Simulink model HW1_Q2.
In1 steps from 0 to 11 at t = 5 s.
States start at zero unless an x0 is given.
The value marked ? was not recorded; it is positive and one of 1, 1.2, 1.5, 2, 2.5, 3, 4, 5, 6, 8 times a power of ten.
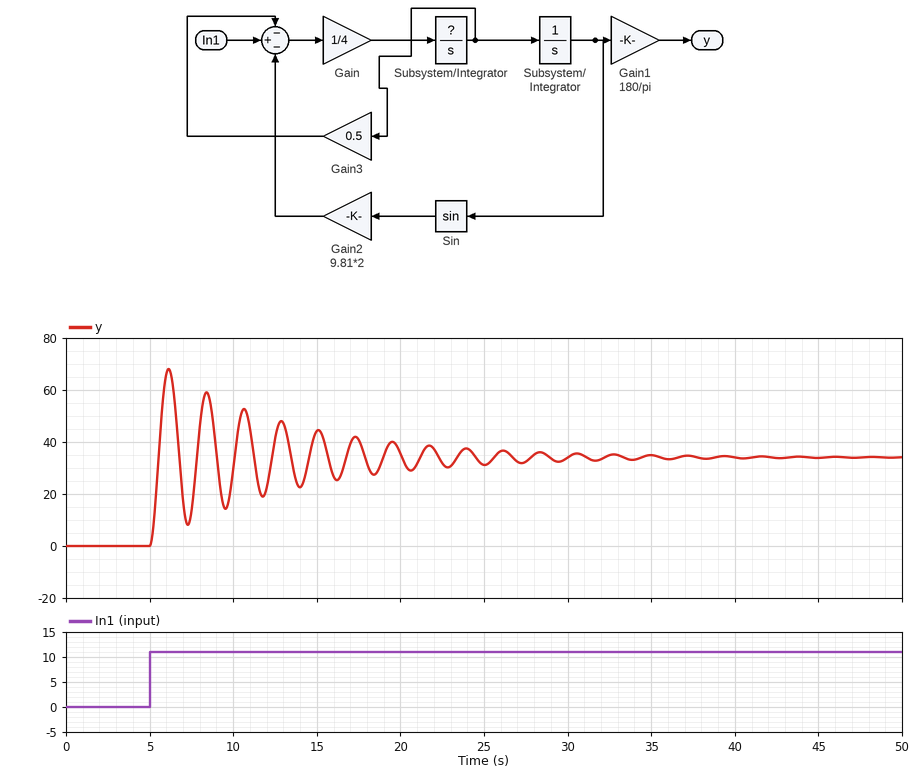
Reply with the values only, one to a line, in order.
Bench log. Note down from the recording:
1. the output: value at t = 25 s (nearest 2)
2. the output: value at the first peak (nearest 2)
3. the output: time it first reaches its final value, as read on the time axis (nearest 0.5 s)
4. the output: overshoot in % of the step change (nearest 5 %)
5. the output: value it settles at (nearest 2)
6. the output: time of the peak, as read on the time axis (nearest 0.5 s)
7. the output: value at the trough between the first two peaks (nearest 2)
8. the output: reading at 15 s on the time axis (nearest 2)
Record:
32
68
5.5 s
100 %
34
6.0 s
8
44
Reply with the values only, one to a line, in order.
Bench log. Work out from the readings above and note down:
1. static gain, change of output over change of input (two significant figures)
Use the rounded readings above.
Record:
3.1
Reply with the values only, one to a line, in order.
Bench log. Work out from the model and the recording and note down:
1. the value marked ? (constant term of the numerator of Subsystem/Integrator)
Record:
2
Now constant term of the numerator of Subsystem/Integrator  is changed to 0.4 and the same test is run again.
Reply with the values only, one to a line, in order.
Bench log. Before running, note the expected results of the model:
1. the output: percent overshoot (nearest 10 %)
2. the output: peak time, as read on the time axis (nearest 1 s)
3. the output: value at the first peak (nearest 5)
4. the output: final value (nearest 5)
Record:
90 %
7 s
65
35
